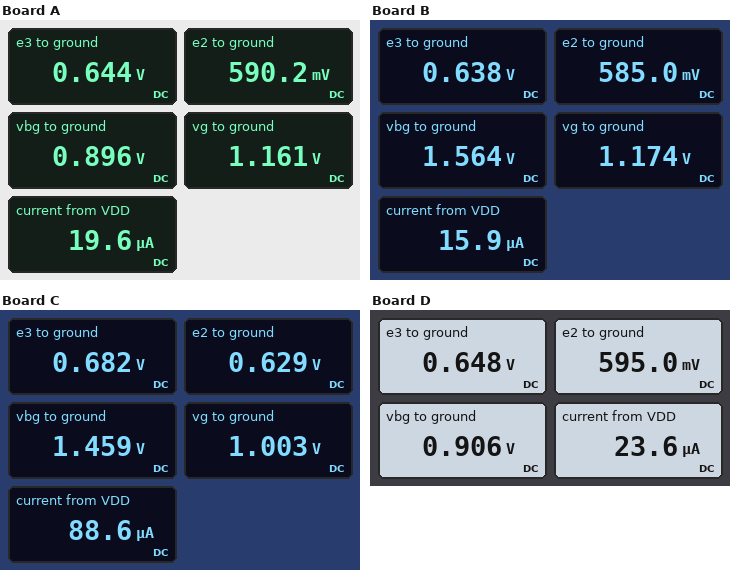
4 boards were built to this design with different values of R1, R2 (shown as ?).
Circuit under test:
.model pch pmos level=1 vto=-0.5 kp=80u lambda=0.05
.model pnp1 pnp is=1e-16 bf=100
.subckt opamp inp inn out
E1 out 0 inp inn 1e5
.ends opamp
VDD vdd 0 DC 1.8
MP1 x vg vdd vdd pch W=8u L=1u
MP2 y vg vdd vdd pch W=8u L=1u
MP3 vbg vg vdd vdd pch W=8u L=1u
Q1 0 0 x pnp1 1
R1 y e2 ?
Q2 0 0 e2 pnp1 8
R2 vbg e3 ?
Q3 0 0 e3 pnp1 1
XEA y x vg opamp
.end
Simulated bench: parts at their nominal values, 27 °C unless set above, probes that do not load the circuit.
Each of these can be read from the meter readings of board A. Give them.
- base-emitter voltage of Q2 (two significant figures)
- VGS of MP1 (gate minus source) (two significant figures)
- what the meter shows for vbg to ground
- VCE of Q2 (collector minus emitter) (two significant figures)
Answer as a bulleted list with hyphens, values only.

- -590 mV
- -640 mV
- 0.896 V
- -590 mV
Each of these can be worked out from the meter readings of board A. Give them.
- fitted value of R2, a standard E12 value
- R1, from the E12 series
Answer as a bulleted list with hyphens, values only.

- 39 kΩ
- 8.2 kΩ
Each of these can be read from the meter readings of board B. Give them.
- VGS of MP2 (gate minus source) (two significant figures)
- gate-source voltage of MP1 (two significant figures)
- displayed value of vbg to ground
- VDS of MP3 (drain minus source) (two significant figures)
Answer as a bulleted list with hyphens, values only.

- -630 mV
- -630 mV
- 1.564 V
- -240 mV
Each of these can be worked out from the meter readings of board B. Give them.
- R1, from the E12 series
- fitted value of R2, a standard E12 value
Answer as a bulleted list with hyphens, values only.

- 10 kΩ
- 180 kΩ
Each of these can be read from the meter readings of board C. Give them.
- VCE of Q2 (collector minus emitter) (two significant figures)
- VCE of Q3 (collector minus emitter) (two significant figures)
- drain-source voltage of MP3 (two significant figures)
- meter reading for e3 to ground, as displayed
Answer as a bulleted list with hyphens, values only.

- -630 mV
- -680 mV
- -340 mV
- 0.682 V
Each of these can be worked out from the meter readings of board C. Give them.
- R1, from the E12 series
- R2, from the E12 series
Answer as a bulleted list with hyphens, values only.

- 1.8 kΩ
- 27 kΩ
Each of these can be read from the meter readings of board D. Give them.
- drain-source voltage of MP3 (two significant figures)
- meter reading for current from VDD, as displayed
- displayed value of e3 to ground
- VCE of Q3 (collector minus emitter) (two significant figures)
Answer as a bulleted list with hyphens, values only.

- -890 mV
- 23.6 µA
- 0.648 V
- -650 mV
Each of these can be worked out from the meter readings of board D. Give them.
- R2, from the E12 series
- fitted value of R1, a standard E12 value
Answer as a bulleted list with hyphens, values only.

- 33 kΩ
- 6.8 kΩ
